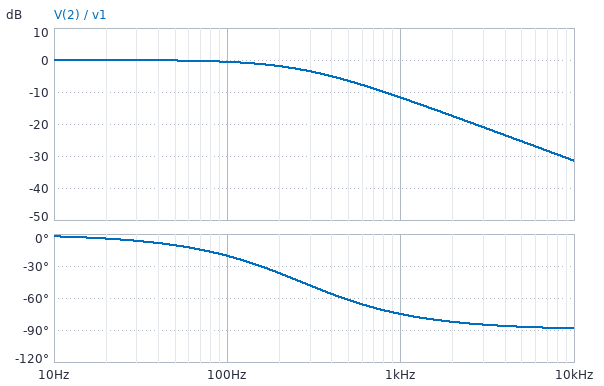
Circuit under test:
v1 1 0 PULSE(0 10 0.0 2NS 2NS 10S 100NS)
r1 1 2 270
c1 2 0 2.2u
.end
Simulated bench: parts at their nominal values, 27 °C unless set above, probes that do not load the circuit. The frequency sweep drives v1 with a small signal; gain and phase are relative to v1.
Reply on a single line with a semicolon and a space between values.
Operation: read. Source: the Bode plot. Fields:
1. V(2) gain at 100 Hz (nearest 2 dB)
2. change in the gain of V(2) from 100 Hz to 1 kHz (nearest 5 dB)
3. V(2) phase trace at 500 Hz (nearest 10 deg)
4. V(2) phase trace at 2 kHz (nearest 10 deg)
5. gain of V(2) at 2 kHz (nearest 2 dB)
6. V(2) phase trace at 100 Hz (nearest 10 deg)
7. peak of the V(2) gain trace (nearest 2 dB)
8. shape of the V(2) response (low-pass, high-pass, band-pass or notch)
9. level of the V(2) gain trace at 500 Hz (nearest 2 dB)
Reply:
0 dB; -10 dB; -60 deg; -80 deg; -18 dB; -20 deg; 0 dB; low-pass; -6 dB
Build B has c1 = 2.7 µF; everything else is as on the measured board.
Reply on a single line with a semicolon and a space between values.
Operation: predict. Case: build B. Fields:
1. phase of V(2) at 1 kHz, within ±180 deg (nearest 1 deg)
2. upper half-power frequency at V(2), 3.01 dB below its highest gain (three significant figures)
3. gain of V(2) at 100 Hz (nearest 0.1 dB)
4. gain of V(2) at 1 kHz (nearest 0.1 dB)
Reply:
-78 deg; 218 Hz; -0.8 dB; -13.4 dB
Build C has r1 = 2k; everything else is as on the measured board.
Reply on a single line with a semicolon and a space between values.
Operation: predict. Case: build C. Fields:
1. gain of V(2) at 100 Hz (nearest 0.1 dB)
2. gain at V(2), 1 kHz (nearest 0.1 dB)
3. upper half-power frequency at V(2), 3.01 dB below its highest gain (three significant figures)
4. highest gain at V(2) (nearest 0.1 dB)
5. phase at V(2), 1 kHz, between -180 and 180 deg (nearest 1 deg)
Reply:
-9.4 dB; -28.8 dB; 36.2 Hz; 0 dB; -88 deg
